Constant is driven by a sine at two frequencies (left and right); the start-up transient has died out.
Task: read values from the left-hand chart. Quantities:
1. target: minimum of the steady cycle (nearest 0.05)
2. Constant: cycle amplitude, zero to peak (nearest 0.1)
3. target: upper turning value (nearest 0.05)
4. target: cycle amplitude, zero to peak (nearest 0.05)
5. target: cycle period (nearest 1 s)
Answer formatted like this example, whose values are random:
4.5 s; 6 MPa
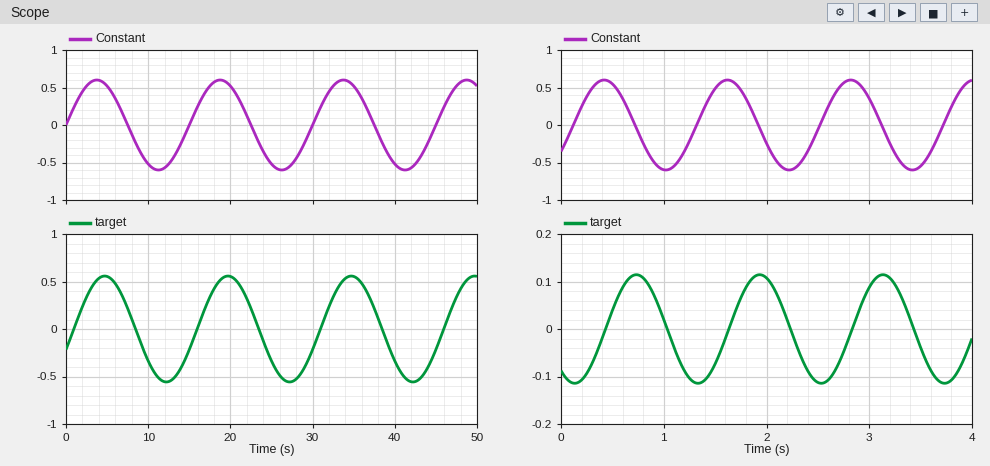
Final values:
-0.55; 0.6; 0.55; 0.55; 15 s
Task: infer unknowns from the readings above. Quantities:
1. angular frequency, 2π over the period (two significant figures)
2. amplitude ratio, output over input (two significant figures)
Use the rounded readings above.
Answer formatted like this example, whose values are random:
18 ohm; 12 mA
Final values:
0.42 rad/s; 0.92
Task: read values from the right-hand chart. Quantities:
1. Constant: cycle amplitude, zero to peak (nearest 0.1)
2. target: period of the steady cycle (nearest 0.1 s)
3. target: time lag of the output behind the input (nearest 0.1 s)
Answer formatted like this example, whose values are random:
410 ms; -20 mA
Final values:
0.6; 1.2 s; 0.3 s
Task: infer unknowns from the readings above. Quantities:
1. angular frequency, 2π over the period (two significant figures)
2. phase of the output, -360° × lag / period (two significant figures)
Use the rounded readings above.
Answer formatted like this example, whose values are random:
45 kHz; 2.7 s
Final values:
5.2 rad/s; -90°
